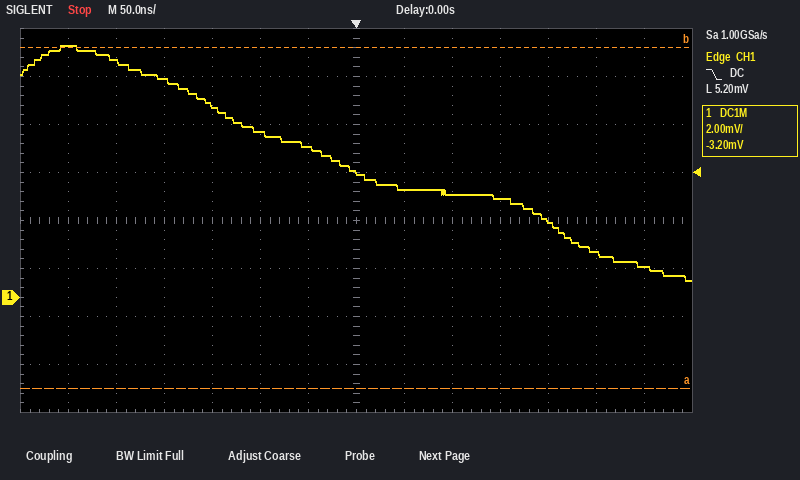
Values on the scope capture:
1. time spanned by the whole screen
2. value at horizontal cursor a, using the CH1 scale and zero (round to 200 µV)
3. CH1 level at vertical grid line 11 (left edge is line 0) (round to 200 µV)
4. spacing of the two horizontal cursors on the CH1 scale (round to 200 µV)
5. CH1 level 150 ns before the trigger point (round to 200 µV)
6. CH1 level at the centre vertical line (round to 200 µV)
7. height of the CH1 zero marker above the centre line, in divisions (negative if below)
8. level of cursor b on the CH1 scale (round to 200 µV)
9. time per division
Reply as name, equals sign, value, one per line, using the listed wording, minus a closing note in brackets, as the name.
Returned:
time spanned by the whole screen = 700 ns
value at horizontal cursor a, using the CH1 scale and zero = -3.8 mV
CH1 level at vertical grid line 11 (left edge is line 0) = 3.2 mV
spacing of the two horizontal cursors on the CH1 scale = 14.2 mV
CH1 level 150 ns before the trigger point = 8.0 mV
CH1 level at the centre vertical line = 5.2 mV
height of the CH1 zero marker above the centre line, in divisions = -1.6 div
level of cursor b on the CH1 scale = 10.4 mV
time per division = 50 ns
